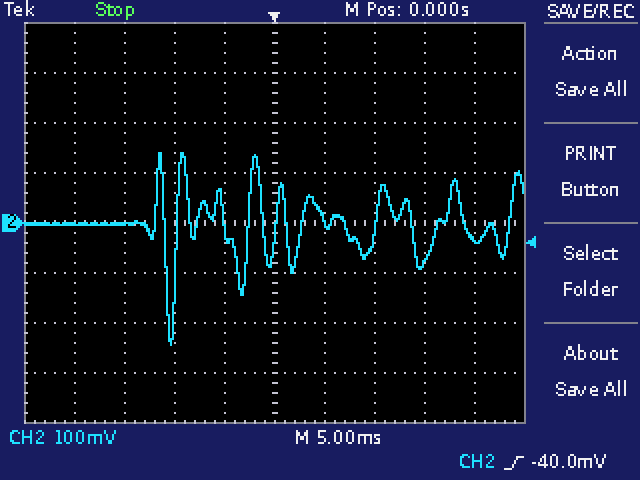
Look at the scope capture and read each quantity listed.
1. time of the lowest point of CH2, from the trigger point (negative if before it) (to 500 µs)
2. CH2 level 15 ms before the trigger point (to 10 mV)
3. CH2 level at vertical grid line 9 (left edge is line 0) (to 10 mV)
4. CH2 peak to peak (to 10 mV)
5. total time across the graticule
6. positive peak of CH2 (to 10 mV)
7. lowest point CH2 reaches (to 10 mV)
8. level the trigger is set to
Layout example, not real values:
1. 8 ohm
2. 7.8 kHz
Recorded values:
1. -10.5 ms
2. 0 mV
3. -30 mV
4. 380 mV
5. 50 ms
6. 140 mV
7. -240 mV
8. -40.0 mV
